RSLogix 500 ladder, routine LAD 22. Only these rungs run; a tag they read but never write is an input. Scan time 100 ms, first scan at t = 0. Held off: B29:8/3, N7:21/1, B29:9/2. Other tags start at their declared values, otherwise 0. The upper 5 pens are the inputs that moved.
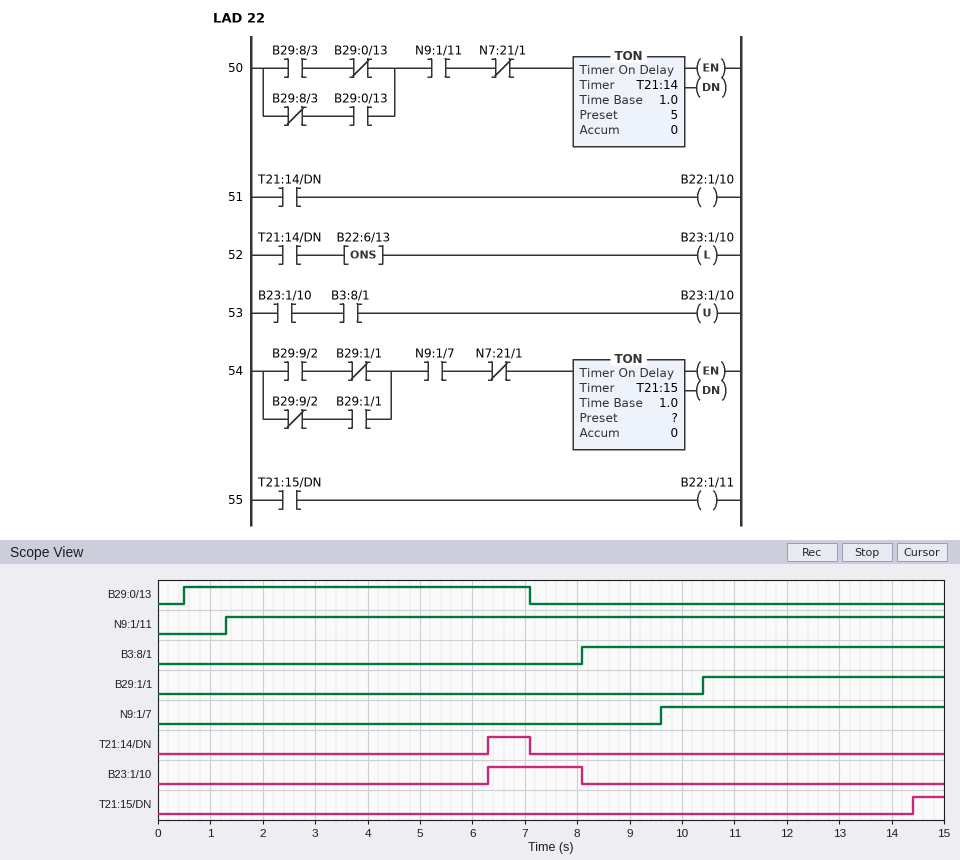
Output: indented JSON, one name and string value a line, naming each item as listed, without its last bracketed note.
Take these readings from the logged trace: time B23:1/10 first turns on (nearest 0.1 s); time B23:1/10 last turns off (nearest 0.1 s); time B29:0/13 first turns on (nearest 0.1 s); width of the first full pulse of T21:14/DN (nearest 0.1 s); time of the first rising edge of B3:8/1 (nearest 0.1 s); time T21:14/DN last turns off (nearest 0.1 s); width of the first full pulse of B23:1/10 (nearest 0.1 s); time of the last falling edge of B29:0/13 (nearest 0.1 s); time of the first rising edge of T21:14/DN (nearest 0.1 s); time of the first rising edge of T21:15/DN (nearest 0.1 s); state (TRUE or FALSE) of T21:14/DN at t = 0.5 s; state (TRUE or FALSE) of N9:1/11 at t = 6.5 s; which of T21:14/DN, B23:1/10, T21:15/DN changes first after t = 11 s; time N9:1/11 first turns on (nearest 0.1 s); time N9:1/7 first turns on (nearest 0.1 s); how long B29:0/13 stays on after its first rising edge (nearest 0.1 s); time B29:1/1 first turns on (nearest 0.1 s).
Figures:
{
  "time B23:1/10 first turns on": "6.3 s",
  "time B23:1/10 last turns off": "8.1 s",
  "time B29:0/13 first turns on": "0.5 s",
  "width of the first full pulse of T21:14/DN": "0.8 s",
  "time of the first rising edge of B3:8/1": "8.1 s",
  "time T21:14/DN last turns off": "7.1 s",
  "width of the first full pulse of B23:1/10": "1.8 s",
  "time of the last falling edge of B29:0/13": "7.1 s",
  "time of the first rising edge of T21:14/DN": "6.3 s",
  "time of the first rising edge of T21:15/DN": "14.4 s",
  "state (TRUE or FALSE) of T21:14/DN at t = 0.5 s": "FALSE",
  "state (TRUE or FALSE) of N9:1/11 at t = 6.5 s": "TRUE",
  "which of T21:14/DN, B23:1/10, T21:15/DN changes first after t = 11 s": "T21:15/DN",
  "time N9:1/11 first turns on": "1.3 s",
  "time N9:1/7 first turns on": "9.6 s",
  "how long B29:0/13 stays on after its first rising edge": "6.6 s",
  "time B29:1/1 first turns on": "10.4 s"
}
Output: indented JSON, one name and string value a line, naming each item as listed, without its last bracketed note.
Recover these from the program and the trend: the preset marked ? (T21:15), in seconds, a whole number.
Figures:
{
  "the preset marked ? (T21:15), in seconds, a whole number": "4 s"
}
